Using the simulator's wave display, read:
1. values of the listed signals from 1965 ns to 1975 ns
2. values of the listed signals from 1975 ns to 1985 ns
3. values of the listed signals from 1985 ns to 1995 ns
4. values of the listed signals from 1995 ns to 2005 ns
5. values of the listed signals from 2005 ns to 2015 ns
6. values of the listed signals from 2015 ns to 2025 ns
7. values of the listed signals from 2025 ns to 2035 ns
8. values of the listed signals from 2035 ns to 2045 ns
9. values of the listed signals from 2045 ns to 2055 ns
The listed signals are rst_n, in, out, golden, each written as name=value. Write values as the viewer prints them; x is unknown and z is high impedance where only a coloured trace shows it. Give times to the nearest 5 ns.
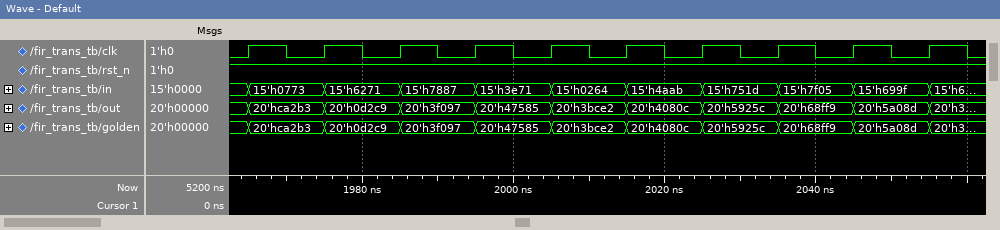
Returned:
rst_n=1, in=15'h0773, out=20'hca2b3, golden=20'hca2b3
rst_n=1, in=15'h6271, out=20'h0d2c9, golden=20'h0d2c9
rst_n=1, in=15'h7887, out=20'h3f097, golden=20'h3f097
rst_n=1, in=15'h3e71, out=20'h47585, golden=20'h47585
rst_n=1, in=15'h0264, out=20'h3bce2, golden=20'h3bce2
rst_n=1, in=15'h4aab, out=20'h4080c, golden=20'h4080c
rst_n=1, in=15'h751d, out=20'h5925c, golden=20'h5925c
rst_n=1, in=15'h7f05, out=20'h68ff9, golden=20'h68ff9
rst_n=1, in=15'h699f, out=20'h5a08d, golden=20'h5a08d
